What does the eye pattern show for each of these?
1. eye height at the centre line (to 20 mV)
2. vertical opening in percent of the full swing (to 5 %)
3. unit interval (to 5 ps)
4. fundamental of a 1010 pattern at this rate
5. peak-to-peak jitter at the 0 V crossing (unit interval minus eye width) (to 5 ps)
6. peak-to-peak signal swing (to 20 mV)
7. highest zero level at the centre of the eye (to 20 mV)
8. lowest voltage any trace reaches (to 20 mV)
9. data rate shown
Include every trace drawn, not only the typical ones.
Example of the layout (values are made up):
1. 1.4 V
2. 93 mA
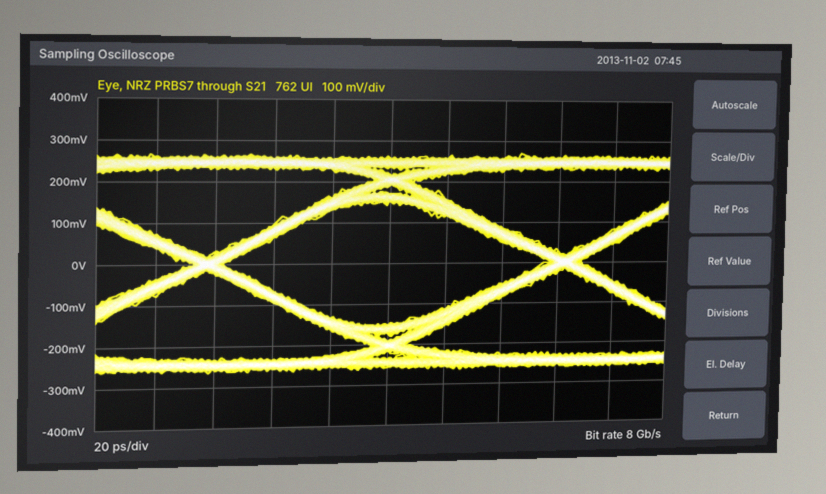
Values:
1. 300 mV
2. 55 %
3. 125 ps
4. 4 GHz
5. 10 ps
6. 540 mV
7. -160 mV
8. -260 mV
9. 8 Gb/s
